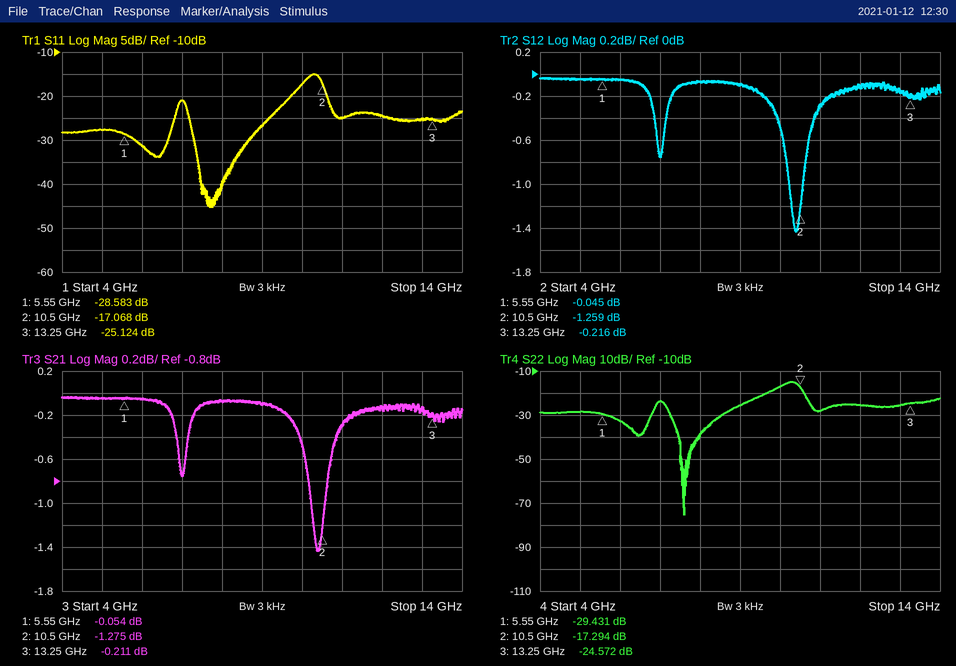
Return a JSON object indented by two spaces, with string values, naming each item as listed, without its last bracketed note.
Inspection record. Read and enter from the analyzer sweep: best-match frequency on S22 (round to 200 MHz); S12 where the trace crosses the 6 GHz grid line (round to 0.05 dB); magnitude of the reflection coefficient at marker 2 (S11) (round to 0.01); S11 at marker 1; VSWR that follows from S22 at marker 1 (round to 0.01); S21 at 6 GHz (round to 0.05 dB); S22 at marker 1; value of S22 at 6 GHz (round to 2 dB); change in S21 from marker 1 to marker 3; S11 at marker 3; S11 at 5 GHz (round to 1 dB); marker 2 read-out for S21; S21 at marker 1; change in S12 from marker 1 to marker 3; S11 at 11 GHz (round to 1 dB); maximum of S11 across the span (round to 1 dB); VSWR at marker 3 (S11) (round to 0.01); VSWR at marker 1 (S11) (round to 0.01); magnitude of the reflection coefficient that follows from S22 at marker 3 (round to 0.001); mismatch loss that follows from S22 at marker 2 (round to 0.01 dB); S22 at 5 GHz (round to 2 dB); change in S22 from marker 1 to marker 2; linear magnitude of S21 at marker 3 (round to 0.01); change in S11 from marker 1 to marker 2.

{
  "best-match frequency on S22": "7.6 GHz",
  "S12 where the trace crosses the 6 GHz grid line": "-0.05 dB",
  "magnitude of the reflection coefficient at marker 2 (S11)": "0.14",
  "S11 at marker 1": "-28.583 dB",
  "VSWR that follows from S22 at marker 1": "1.07",
  "S21 at 6 GHz": "-0.05 dB",
  "S22 at marker 1": "-29.431 dB",
  "value of S22 at 6 GHz": "-32 dB",
  "change in S21 from marker 1 to marker 3": "-0.157 dB",
  "S11 at marker 3": "-25.124 dB",
  "S11 at 5 GHz": "-28 dB",
  "marker 2 read-out for S21": "-1.275 dB",
  "S21 at marker 1": "-0.054 dB",
  "change in S12 from marker 1 to marker 3": "-0.171 dB",
  "S11 at 11 GHz": "-25 dB",
  "maximum of S11 across the span": "-15 dB",
  "VSWR at marker 3 (S11)": "1.12",
  "VSWR at marker 1 (S11)": "1.08",
  "magnitude of the reflection coefficient that follows from S22 at marker 3": "0.059",
  "mismatch loss that follows from S22 at marker 2": "0.08 dB",
  "S22 at 5 GHz": "-28 dB",
  "change in S22 from marker 1 to marker 2": "12.137 dB",
  "linear magnitude of S21 at marker 3": "0.98",
  "change in S11 from marker 1 to marker 2": "11.515 dB"
}
